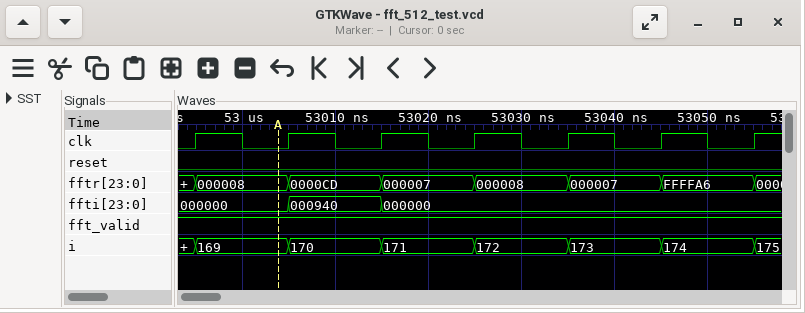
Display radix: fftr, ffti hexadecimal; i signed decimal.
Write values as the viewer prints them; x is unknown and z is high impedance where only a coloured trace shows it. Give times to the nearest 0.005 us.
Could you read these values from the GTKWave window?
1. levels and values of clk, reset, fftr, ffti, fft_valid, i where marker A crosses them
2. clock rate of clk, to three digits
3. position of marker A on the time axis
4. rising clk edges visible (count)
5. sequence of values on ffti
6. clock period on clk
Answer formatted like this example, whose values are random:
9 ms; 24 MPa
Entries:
clk=0, reset=0, fftr=000008, ffti=000000, fft_valid=1, i=169; 100 MHz; 53.005 us; 7; 000000, 000940, 000000; 0.01 us
